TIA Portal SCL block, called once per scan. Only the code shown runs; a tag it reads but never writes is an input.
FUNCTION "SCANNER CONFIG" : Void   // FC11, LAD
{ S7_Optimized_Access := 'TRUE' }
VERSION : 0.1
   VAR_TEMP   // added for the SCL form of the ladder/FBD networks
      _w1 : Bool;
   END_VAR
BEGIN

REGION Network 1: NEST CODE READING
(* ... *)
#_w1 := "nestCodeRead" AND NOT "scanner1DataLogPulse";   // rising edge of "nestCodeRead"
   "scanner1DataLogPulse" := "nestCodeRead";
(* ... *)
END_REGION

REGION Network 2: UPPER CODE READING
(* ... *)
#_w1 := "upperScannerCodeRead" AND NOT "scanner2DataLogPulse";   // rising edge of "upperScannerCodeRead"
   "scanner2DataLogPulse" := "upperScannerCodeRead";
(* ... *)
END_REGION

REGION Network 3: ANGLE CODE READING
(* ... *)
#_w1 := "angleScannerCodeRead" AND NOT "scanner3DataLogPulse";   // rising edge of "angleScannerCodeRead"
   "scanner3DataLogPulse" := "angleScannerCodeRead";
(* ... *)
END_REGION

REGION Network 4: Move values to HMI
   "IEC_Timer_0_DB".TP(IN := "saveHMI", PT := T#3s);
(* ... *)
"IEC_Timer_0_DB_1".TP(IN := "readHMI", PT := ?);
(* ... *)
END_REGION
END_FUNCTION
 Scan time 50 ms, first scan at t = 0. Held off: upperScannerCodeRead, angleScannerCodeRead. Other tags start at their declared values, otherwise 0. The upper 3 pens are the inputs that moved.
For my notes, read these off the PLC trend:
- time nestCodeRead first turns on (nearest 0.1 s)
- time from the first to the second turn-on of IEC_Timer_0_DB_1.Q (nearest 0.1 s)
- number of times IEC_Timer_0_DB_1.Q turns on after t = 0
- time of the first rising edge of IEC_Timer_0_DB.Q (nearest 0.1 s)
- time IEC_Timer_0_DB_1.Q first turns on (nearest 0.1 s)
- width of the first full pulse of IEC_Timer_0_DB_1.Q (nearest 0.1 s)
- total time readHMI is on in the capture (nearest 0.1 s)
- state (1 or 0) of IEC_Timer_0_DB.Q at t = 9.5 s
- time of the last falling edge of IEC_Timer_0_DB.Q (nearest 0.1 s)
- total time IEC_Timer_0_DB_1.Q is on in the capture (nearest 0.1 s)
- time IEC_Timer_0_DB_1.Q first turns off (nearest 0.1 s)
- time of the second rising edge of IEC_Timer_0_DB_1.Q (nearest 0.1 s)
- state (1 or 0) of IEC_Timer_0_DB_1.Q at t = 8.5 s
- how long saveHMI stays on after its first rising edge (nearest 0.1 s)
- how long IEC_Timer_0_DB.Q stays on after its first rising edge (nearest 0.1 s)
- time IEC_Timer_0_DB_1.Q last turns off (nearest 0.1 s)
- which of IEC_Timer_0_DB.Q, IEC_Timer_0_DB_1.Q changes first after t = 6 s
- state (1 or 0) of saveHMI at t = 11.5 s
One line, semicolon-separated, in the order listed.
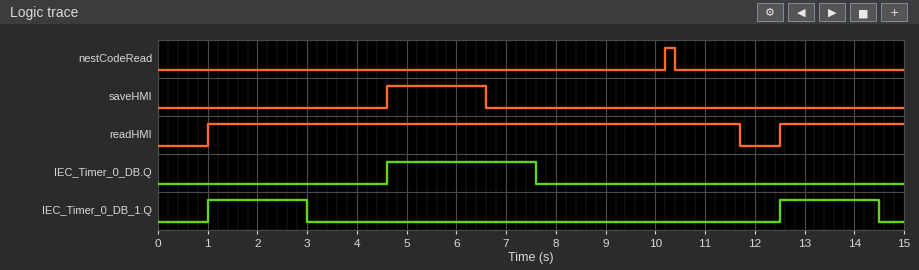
10.2 s; 11.5 s; 2; 4.6 s; 1.0 s; 2.0 s; 13.2 s; 0; 7.6 s; 4.0 s; 3.0 s; 12.5 s; 0; 2.0 s; 3.0 s; 14.5 s; IEC_Timer_0_DB.Q; 0
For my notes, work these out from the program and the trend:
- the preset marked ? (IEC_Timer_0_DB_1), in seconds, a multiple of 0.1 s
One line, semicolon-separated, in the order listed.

2.0 s
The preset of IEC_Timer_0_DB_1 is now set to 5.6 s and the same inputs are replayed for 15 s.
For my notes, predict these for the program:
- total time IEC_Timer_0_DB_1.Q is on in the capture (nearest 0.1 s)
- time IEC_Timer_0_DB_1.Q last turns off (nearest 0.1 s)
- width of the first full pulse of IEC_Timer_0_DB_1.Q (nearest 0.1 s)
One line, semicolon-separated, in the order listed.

8.1 s; 6.6 s; 5.6 s
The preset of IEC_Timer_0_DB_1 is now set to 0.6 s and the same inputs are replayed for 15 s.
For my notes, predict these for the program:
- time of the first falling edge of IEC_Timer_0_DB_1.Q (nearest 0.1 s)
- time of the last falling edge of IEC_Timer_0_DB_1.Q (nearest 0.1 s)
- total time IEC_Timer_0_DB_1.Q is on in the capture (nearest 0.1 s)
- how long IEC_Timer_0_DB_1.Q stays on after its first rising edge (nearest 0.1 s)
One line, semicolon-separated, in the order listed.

1.6 s; 13.1 s; 1.2 s; 0.6 s
